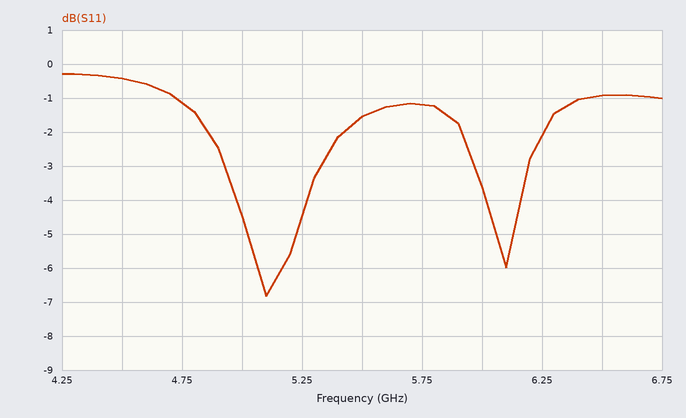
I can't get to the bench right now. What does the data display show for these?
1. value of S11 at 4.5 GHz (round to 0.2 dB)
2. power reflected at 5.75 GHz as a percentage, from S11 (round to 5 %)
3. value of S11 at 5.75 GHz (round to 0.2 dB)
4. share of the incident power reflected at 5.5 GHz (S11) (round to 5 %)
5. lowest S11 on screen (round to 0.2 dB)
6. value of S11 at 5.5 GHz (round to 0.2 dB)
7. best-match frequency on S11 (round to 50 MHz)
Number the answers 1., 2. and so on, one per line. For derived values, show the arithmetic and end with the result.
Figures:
1. -0.4 dB
2. 10^(-1.2/10) ≈ 75.9 %, so 75 % to the nearest 5 %
3. -1.2 dB
4. 10^(-1.6/10) ≈ 69.2 %, so 70 % to the nearest 5 %
5. -6.8 dB
6. -1.6 dB
7. 5.10 GHz
